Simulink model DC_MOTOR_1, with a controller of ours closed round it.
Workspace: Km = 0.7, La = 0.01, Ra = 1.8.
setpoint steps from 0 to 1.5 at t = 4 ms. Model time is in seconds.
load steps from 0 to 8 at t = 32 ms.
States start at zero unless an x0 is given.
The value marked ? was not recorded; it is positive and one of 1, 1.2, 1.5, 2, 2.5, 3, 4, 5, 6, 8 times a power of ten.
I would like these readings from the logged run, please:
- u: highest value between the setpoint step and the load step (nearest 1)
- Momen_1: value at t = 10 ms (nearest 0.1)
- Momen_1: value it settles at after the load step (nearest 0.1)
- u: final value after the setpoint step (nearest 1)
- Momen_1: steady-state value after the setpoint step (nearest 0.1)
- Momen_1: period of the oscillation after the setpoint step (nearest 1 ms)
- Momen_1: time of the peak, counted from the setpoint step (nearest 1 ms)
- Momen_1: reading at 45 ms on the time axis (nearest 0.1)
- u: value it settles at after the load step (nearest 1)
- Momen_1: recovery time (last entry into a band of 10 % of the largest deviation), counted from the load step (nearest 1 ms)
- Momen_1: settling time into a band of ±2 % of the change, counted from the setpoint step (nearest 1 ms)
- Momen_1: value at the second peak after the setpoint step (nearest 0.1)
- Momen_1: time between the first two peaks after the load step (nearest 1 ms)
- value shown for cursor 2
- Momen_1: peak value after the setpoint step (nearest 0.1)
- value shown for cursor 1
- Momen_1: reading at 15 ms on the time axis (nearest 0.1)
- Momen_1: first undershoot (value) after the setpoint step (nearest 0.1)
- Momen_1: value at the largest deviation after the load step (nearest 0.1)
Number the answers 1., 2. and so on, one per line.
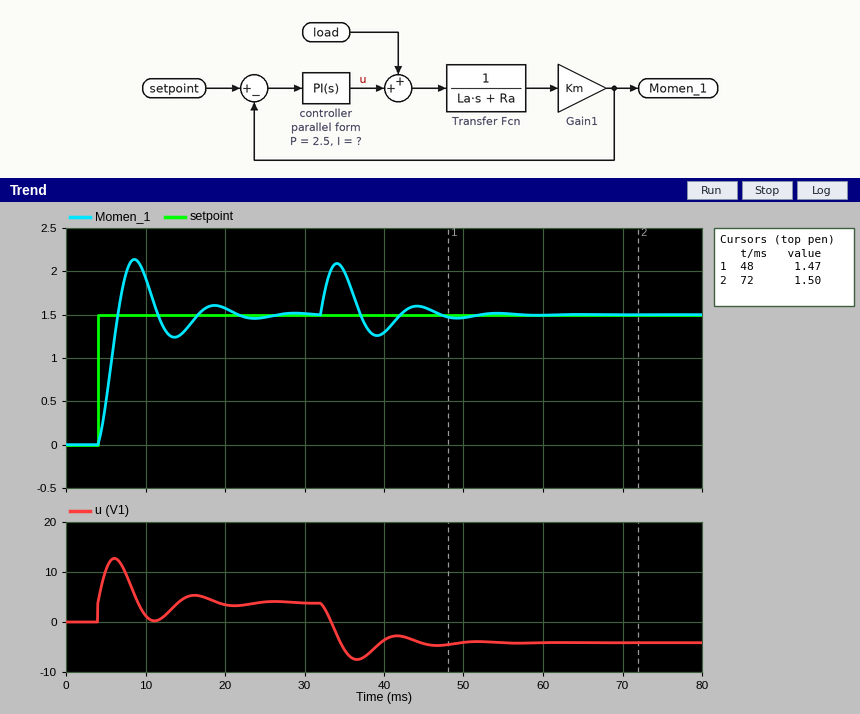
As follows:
1. 13
2. 1.9
3. 1.5
4. 4
5. 1.5
6. 10 ms
7. 5 ms
8. 1.6
9. -4
10. 14 ms
11. 21 ms
12. 1.6
13. 10 ms
14. 1.50
15. 2.1
16. 1.47
17. 1.3
18. 1.2
19. 2.1
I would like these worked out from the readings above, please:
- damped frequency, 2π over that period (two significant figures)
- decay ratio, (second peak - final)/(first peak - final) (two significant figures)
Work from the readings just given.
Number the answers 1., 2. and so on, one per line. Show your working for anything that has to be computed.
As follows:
1. 2π / 10 = 0.63 rad/ms
2. (1.6 - 1.5) / (2.1 - 1.5) = 0.17
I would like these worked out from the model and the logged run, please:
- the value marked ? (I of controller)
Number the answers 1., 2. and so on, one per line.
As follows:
1. 6000
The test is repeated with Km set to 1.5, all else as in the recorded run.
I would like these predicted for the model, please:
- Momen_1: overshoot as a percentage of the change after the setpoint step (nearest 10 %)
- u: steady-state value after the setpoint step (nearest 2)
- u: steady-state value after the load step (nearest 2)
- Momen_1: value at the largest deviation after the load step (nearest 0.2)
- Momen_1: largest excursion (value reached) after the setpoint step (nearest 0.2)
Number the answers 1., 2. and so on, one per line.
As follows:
1. 40 %
2. 2
3. -6
4. 2.4
5. 2.2
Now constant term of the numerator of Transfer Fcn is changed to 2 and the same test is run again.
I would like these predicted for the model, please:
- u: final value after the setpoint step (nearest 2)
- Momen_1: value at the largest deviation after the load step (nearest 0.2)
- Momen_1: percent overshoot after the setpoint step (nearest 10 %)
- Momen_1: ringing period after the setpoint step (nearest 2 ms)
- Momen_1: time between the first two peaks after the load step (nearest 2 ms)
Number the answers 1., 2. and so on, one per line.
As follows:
1. 2
2. 2.4
3. 40 %
4. 8 ms
5. 8 ms
